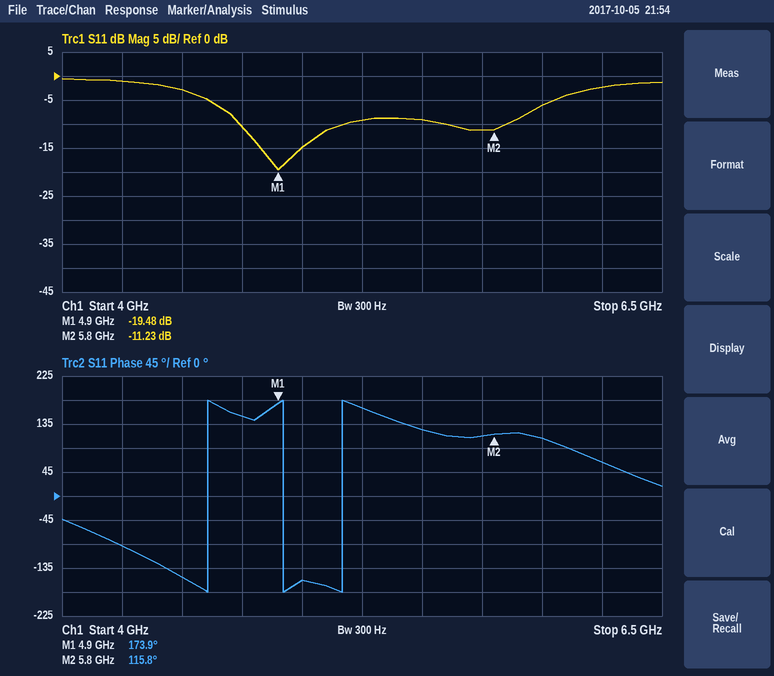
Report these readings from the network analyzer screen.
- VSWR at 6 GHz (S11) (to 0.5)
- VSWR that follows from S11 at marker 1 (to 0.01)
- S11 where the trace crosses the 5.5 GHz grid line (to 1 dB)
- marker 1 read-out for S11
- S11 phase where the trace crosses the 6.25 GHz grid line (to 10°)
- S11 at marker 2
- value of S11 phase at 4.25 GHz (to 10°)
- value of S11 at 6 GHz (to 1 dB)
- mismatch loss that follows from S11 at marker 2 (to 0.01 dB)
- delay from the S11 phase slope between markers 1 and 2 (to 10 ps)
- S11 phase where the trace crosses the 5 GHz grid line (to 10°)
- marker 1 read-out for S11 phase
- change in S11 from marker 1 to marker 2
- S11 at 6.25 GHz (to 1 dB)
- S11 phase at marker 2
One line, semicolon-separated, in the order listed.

3.0; 1.24; -9 dB; -19.48 dB; 60°; -11.23 dB; -90°; -6 dB; 0.34 dB; 180 ps; -160°; 173.9°; 8.25 dB; -2 dB; 115.8°
